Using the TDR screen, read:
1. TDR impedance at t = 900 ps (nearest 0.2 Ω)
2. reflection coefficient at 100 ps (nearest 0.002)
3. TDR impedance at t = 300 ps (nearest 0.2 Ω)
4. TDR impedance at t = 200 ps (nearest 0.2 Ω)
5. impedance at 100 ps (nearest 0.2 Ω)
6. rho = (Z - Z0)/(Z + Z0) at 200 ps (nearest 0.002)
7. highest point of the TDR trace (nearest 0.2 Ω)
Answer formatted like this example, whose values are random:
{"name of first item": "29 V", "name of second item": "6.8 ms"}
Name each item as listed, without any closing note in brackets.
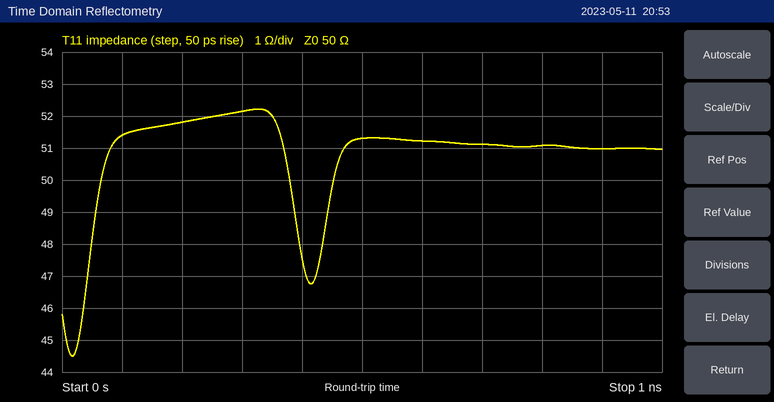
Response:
{"TDR impedance at t = 900 ps": "51.0 Ω", "reflection coefficient at 100 ps": "+0.014", "TDR impedance at t = 300 ps": "52.2 Ω", "TDR impedance at t = 200 ps": "51.8 Ω", "impedance at 100 ps": "51.4 Ω", "rho = (Z - Z0)/(Z + Z0) at 200 ps": "+0.018", "highest point of the TDR trace": "52.2 Ω"}
